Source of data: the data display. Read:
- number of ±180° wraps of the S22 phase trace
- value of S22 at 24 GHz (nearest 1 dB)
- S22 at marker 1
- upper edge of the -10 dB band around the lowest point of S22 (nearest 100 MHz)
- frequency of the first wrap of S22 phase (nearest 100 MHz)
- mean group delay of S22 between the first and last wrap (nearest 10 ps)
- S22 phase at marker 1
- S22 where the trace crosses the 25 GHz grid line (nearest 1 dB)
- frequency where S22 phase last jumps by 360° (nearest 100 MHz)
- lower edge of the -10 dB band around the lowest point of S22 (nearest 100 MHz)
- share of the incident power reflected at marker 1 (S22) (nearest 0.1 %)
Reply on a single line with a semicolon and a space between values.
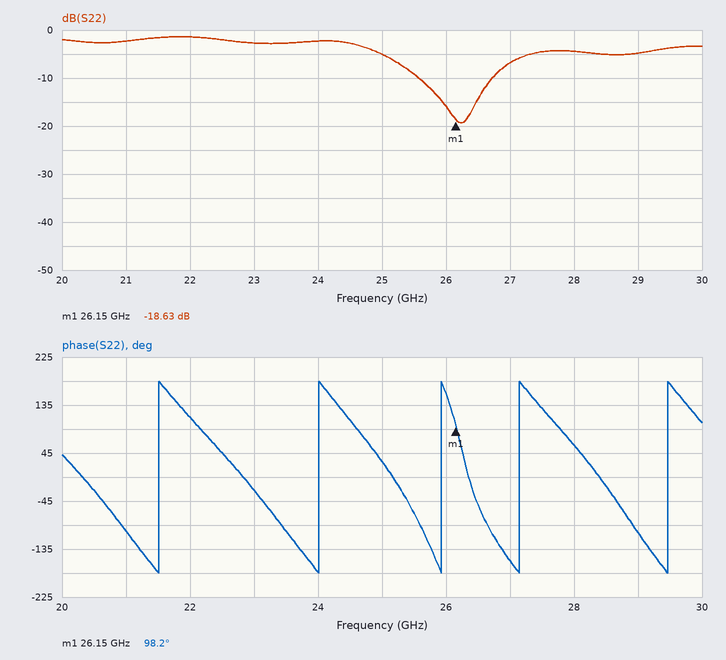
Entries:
5; -2 dB; -18.63 dB; 26.7 GHz; 21.5 GHz; 500 ps; 98.2°; -5 dB; 29.5 GHz; 25.6 GHz; 1.4 %
